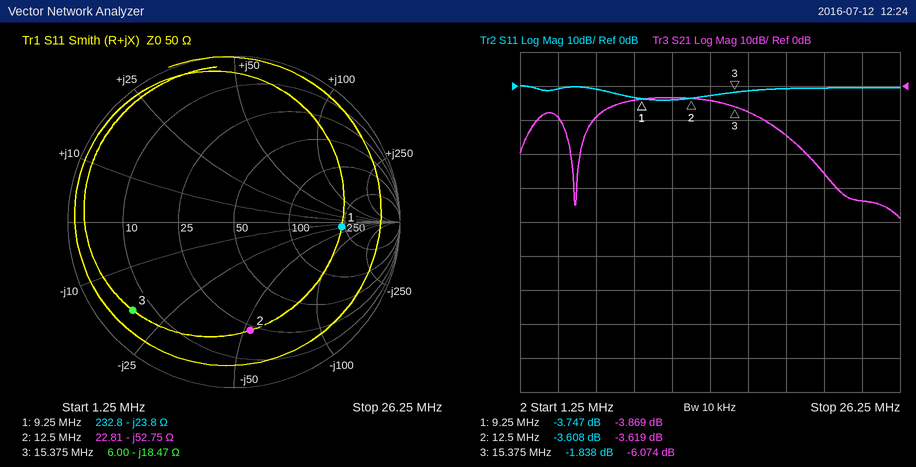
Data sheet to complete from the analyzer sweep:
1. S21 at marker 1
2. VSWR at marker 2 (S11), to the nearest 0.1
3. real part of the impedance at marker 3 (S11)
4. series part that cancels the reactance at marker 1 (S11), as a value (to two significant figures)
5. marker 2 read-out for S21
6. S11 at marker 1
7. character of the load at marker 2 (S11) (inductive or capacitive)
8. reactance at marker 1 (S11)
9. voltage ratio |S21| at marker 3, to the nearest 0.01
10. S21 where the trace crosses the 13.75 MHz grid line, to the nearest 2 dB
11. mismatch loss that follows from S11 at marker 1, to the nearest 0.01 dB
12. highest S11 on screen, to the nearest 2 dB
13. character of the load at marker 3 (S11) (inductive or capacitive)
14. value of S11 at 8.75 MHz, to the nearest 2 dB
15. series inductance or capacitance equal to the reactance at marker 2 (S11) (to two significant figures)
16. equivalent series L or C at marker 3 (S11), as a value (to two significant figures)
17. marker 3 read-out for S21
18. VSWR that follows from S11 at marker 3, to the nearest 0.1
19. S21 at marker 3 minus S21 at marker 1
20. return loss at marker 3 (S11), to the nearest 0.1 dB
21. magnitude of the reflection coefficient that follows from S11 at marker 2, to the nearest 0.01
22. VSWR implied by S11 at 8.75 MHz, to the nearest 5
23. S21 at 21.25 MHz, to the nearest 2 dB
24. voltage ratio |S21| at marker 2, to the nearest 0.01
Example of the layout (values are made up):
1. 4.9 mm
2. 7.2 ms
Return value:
1. -3.869 dB
2. 4.9
3. 6.00 Ω
4. 410 nH
5. -3.619 dB
6. -3.747 dB
7. capacitive
8. -23.8 Ω
9. 0.50
10. -4 dB
11. 2.38 dB
12. 0 dB
13. capacitive
14. -4 dB
15. 240 pF
16. 560 pF
17. -6.074 dB
18. 9.5
19. -2.205 dB
20. 1.8 dB
21. 0.66
22. 5
23. -26 dB
24. 0.66
